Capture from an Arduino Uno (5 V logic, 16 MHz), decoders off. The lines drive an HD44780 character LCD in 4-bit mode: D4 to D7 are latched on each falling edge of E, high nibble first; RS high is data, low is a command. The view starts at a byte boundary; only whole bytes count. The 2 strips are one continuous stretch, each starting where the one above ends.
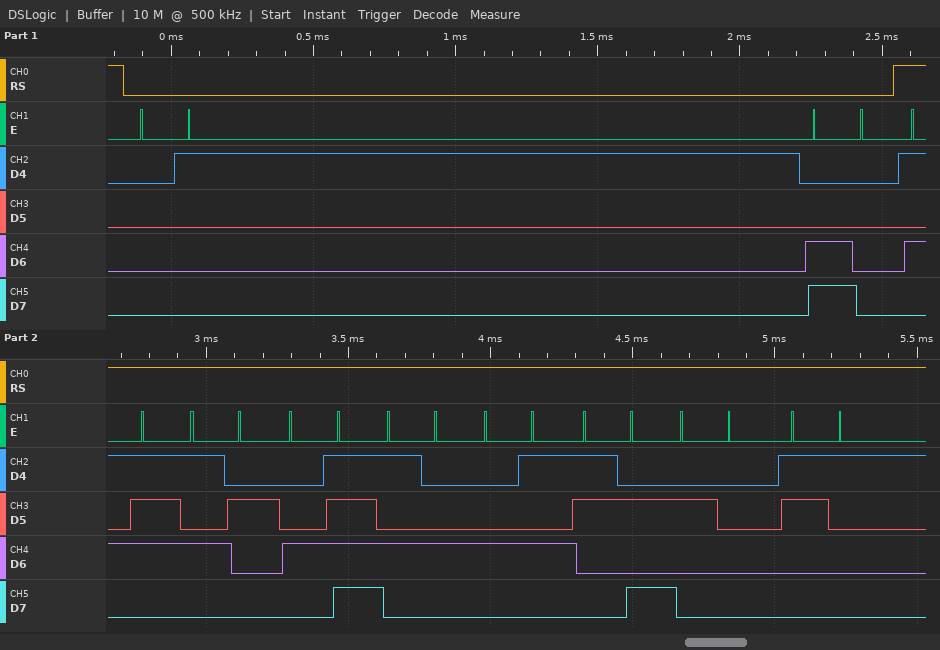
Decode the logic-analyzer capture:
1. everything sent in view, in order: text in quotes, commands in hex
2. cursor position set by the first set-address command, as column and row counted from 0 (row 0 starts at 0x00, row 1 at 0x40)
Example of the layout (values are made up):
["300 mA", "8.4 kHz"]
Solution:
["0x01 0xC0 \"WROTE: 1\"", "column 0, row 1"]
